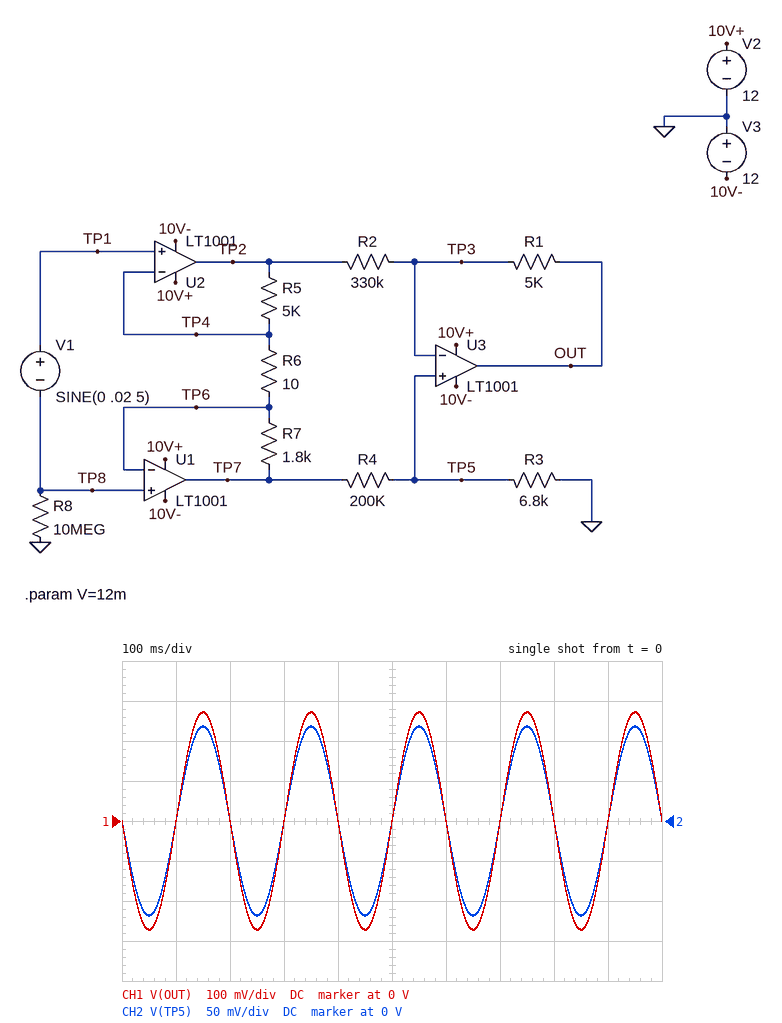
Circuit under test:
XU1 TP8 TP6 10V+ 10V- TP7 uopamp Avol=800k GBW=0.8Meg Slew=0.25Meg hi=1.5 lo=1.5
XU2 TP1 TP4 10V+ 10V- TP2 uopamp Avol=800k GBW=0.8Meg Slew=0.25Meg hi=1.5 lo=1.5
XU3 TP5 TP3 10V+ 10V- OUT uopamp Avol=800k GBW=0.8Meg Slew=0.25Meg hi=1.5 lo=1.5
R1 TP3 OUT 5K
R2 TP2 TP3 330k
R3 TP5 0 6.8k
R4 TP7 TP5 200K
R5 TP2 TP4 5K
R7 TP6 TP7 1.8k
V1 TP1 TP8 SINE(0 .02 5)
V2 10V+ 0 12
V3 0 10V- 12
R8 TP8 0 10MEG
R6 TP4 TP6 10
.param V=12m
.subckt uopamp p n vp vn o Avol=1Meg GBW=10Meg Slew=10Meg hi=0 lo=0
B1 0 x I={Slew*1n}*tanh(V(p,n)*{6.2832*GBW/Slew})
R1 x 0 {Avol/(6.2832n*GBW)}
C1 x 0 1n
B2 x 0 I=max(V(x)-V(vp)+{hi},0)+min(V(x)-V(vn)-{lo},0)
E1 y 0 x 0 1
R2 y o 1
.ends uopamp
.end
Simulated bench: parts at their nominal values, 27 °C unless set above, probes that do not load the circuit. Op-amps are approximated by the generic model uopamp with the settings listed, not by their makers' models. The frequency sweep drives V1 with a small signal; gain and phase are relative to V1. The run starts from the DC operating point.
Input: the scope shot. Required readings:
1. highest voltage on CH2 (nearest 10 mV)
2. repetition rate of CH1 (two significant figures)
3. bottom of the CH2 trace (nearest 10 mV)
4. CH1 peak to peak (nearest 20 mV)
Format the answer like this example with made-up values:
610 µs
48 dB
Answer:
120 mV
5.0 Hz
-120 mV
540 mV
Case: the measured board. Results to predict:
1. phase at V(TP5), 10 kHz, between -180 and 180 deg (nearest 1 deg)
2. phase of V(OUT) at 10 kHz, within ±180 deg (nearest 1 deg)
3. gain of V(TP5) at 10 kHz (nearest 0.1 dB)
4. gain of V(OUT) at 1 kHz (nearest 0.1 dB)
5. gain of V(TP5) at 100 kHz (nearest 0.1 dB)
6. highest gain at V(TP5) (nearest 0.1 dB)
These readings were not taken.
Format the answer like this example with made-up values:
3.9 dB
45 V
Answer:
96 deg
96 deg
-3.2 dB
20.3 dB
-23.2 dB
15.4 dB
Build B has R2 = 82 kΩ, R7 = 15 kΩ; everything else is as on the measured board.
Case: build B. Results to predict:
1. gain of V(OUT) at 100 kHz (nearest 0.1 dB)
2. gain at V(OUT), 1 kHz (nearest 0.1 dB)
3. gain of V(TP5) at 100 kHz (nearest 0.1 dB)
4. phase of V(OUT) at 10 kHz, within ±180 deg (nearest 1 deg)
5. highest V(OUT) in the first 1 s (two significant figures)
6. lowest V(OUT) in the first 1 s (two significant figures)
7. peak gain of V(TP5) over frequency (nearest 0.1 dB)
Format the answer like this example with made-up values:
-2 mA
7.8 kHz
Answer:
-9.6 dB
29.8 dB
-14.2 dB
92 deg
580 mV
-580 mV
33.8 dB
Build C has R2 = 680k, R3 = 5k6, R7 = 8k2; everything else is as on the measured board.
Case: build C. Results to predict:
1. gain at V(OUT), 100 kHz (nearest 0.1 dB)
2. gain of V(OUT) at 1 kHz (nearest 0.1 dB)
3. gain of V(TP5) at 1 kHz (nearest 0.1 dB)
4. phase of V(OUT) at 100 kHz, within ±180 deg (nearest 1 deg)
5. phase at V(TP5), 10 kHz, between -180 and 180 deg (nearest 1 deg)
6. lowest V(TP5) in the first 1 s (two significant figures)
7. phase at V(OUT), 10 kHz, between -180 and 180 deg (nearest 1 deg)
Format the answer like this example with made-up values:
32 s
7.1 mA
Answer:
-16.1 dB
22.6 dB
21.3 dB
79 deg
93 deg
-290 mV
92 deg
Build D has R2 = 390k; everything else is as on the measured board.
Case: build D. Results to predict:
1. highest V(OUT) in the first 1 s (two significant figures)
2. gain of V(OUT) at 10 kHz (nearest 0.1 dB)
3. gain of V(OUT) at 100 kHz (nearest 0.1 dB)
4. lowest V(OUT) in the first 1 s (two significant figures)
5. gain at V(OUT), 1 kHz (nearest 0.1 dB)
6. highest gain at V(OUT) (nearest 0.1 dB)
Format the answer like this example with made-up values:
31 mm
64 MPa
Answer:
250 mV
3.2 dB
-16.8 dB
-250 mV
19.5 dB
21.9 dB
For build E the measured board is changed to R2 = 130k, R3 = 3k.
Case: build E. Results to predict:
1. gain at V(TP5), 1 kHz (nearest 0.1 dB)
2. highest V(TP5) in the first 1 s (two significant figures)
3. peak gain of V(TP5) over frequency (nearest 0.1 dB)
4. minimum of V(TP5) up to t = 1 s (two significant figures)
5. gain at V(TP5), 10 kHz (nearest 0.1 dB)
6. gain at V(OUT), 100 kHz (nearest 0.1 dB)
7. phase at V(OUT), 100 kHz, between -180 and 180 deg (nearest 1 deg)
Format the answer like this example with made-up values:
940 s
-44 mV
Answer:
6.1 dB
53 mV
8.5 dB
-53 mV
-10.2 dB
-11.8 dB
85 deg
